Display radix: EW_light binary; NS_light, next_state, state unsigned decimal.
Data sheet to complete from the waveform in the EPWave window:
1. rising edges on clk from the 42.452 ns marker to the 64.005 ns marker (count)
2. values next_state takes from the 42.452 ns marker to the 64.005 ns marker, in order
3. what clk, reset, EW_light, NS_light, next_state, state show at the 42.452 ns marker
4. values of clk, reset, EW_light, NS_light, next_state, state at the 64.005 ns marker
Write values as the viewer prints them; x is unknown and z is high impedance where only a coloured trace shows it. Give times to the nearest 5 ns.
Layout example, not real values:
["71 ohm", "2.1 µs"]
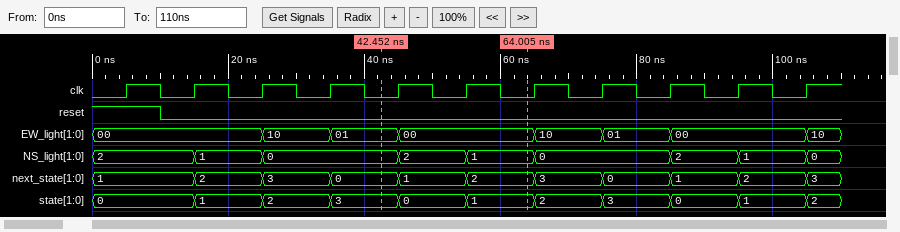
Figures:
["2", "0, 1, 2", "clk=0, reset=0, EW_light=01, NS_light=0, next_state=0, state=3", "clk=0, reset=0, EW_light=00, NS_light=1, next_state=2, state=1"]
